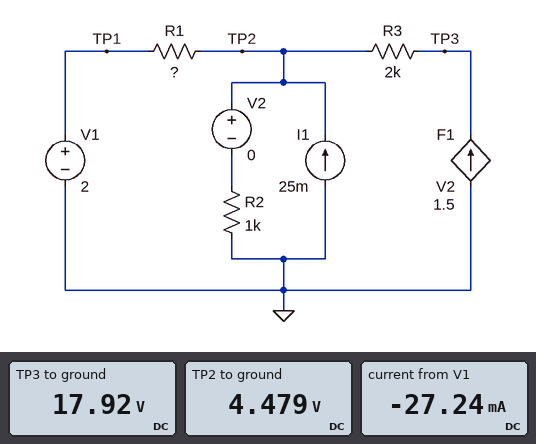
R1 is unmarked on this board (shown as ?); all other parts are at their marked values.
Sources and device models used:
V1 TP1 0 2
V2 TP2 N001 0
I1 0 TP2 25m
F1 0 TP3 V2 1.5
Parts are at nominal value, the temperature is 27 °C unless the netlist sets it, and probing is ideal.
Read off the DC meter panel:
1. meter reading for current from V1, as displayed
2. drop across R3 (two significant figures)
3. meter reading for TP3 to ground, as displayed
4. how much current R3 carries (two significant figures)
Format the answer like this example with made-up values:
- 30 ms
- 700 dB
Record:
- -27.24 mA
- 13 V
- 17.92 V
- 6.7 mA
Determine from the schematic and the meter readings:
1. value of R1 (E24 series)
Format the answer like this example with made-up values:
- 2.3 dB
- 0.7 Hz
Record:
- 91 Ω
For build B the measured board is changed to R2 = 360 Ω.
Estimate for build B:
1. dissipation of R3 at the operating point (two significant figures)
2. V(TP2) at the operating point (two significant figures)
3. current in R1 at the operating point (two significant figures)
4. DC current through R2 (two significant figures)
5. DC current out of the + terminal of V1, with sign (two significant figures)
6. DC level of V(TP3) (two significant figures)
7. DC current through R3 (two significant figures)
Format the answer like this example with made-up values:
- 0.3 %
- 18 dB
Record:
- 830 mW
- 4.9 V
- 32 mA
- 14 mA
- -32 mA
- 46 V
- 20 mA
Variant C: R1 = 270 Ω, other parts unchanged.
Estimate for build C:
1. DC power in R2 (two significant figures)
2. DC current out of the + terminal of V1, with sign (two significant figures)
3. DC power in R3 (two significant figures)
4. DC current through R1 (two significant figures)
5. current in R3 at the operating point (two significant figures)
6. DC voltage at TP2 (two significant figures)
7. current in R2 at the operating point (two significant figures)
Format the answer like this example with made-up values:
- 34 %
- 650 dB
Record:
- 100 mW
- -30 mA
- 460 mW
- 30 mA
- 15 mA
- 10 V
- 10 mA
